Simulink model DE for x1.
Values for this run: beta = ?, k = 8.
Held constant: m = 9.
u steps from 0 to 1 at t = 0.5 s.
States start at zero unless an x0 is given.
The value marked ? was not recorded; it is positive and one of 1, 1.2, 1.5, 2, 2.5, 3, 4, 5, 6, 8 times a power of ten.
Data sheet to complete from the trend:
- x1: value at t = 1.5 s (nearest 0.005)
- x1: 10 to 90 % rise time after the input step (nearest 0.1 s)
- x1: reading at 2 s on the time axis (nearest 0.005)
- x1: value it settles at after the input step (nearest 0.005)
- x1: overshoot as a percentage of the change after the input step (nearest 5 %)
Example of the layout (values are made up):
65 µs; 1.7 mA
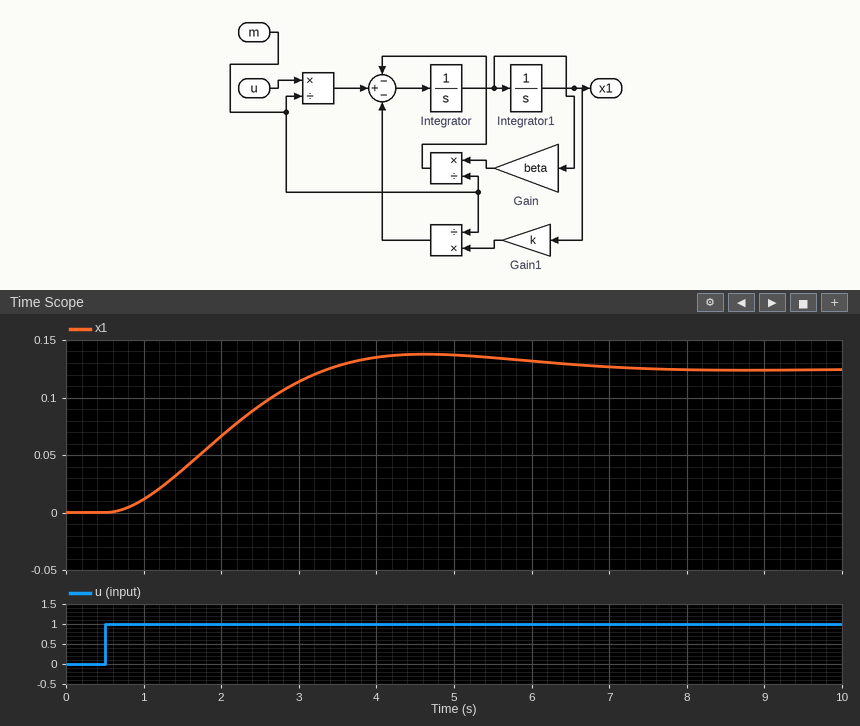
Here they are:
0.035; 1.9 s; 0.065; 0.125; 10 %
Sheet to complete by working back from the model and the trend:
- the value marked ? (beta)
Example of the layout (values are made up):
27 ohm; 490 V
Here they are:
10
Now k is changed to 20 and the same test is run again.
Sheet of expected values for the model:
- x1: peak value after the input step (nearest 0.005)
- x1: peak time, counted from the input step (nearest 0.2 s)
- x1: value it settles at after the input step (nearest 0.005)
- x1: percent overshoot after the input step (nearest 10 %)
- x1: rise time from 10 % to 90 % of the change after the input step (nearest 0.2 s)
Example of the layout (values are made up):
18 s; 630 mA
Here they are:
0.065; 2.2 s; 0.050; 30 %; 1.0 s
